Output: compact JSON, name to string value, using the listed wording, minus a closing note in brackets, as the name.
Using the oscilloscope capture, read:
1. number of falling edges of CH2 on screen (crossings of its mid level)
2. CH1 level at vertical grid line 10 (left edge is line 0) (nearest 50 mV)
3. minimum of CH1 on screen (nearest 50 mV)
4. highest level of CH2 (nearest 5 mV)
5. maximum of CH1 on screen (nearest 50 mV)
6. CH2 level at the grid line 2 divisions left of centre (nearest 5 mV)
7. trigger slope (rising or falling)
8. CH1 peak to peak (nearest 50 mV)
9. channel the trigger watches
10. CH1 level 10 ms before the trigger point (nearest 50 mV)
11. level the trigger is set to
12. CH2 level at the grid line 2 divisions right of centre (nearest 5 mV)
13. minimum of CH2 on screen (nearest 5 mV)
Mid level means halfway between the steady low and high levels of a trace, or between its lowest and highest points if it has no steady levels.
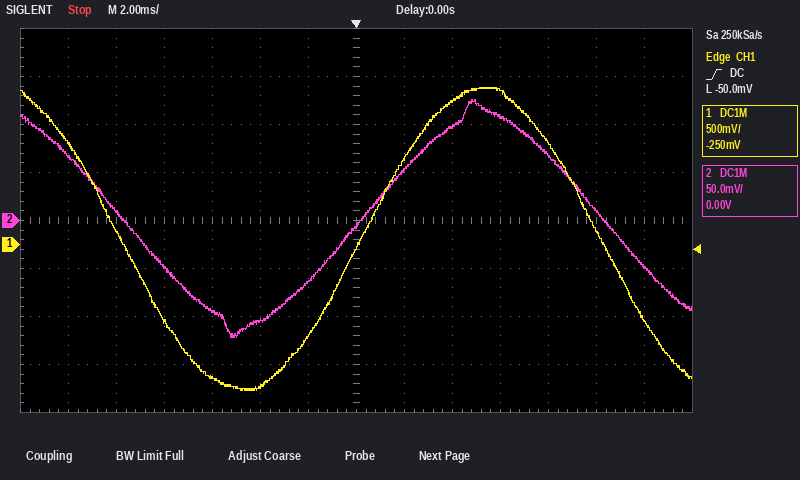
{"number of falling edges of CH2 on screen": "2", "CH1 level at vertical grid line 10 (left edge is line 0)": "1.60 V", "minimum of CH1 on screen": "-1.50 V", "highest level of CH2": "125 mV", "maximum of CH1 on screen": "1.65 V", "CH2 level at the grid line 2 divisions left of centre": "-105 mV", "trigger slope": "rising", "CH1 peak to peak": "3.15 V", "channel the trigger watches": "CH1", "CH1 level 10 ms before the trigger point": "150 mV", "level the trigger is set to": "-50.0 mV", "CH2 level at the grid line 2 divisions right of centre": "100 mV", "minimum of CH2 on screen": "-120 mV"}
